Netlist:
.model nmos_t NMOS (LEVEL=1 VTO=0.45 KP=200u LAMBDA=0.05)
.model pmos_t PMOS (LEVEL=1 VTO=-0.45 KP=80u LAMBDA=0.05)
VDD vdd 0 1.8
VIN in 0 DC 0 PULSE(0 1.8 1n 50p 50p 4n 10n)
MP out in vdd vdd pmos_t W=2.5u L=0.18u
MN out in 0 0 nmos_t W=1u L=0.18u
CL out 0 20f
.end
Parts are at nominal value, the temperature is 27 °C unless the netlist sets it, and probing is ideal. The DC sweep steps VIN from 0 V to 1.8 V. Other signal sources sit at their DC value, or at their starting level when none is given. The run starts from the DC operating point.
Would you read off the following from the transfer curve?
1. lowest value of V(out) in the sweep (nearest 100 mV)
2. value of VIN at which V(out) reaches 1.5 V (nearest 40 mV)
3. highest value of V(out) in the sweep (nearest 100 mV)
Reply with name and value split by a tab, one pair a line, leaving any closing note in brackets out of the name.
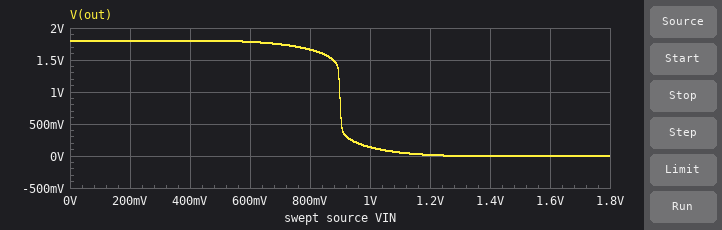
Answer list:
lowest value of V(out) in the sweep	0 V
value of VIN at which V(out) reaches 1.5 V	880 mV
highest value of V(out) in the sweep	1.8 V
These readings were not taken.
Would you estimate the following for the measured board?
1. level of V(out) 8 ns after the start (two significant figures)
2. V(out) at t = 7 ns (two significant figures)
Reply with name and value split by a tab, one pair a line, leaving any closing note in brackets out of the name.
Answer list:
level of V(out) 8 ns after the start	1.8 V
V(out) at t = 7 ns	1.8 V
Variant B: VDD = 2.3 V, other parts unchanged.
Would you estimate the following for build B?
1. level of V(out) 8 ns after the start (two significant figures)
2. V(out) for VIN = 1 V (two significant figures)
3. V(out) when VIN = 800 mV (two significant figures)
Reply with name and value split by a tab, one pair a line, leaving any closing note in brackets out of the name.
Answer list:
level of V(out) 8 ns after the start	2.3 V
V(out) for VIN = 1 V	2.1 V
V(out) when VIN = 800 mV	2.2 V
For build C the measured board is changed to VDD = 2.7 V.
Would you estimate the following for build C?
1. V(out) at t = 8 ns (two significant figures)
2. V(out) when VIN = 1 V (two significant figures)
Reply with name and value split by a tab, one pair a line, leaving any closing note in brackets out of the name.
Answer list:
V(out) at t = 8 ns	2.7 V
V(out) when VIN = 1 V	2.6 V
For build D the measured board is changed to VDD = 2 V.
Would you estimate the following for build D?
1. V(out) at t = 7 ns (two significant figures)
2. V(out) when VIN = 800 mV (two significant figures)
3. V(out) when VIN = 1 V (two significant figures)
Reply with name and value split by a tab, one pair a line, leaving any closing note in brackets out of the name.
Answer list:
V(out) at t = 7 ns	2.0 V
V(out) when VIN = 800 mV	1.9 V
V(out) when VIN = 1 V	1.0 V
